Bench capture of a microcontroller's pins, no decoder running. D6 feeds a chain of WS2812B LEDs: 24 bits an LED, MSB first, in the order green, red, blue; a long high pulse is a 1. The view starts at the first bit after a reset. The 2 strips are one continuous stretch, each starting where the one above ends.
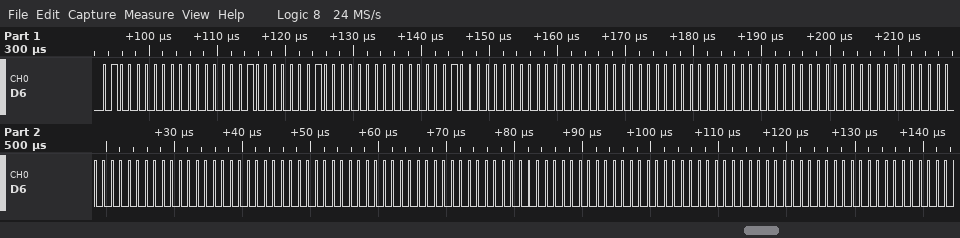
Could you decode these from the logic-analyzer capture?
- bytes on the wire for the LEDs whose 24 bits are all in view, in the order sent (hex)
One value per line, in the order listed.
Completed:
40 00 40 40 00 40 00 00 00 00 00 00 00 00 00 00 00 00 00 00 00 00 00 00
